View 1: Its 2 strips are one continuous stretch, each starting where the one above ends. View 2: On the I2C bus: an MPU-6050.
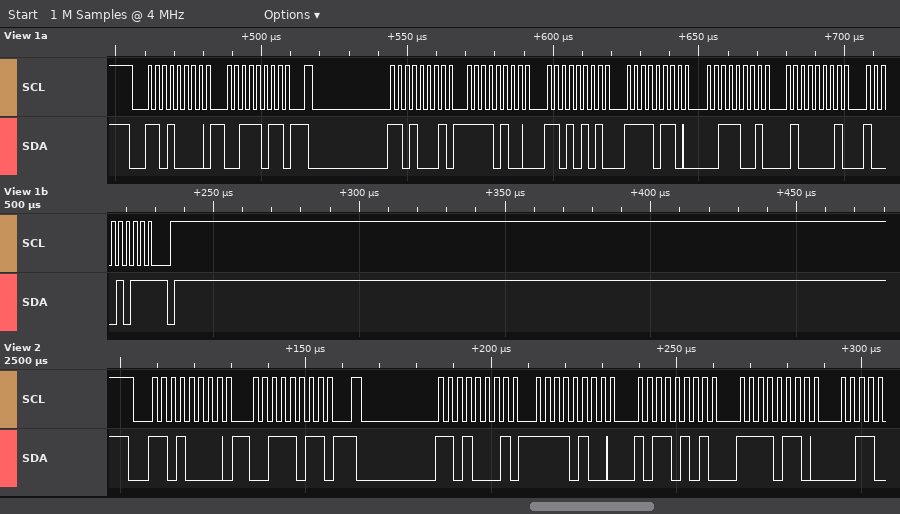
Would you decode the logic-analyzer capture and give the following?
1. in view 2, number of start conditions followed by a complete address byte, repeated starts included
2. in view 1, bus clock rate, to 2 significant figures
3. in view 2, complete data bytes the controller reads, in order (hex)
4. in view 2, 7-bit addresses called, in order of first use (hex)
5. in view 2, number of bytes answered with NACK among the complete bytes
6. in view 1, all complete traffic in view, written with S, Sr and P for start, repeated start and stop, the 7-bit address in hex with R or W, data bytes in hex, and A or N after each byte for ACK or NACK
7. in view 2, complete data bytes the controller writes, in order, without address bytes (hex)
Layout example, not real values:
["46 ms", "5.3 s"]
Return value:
["2", "400 kHz", "F4 B5 F6", "0x68", "0", "S 68W A 3B A Sr 68R A F4 A D5 A F6 A 39 A 41 A 8B N P", "3B"]
